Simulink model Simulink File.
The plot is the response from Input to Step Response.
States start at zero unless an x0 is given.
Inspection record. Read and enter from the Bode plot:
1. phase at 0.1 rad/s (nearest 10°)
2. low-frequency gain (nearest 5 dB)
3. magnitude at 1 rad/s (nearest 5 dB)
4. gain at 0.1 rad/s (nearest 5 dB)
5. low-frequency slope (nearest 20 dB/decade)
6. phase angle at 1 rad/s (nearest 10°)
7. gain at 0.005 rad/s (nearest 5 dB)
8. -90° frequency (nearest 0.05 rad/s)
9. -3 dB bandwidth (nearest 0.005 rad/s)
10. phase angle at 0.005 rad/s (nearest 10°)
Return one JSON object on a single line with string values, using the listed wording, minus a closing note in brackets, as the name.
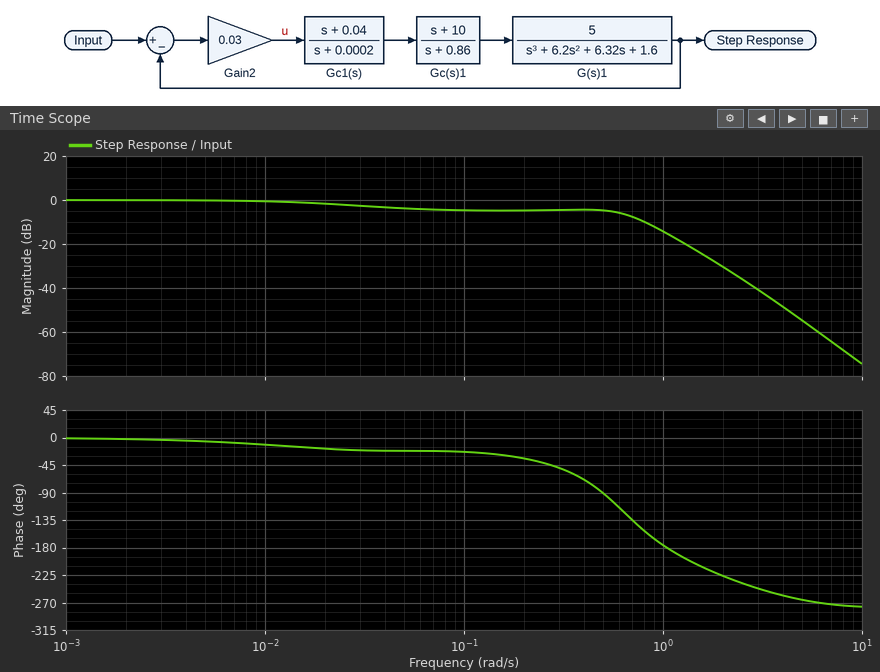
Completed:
{"phase at 0.1 rad/s": "-20°", "low-frequency gain": "0 dB", "magnitude at 1 rad/s": "-15 dB", "gain at 0.1 rad/s": "-5 dB", "low-frequency slope": "0 dB/decade", "phase angle at 1 rad/s": "-180°", "gain at 0.005 rad/s": "0 dB", "-90° frequency": "0.50 rad/s", "-3 dB bandwidth": "0.035 rad/s", "phase angle at 0.005 rad/s": "-10°"}
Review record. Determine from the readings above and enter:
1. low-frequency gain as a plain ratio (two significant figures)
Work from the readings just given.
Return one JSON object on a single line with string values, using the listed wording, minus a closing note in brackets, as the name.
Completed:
{"low-frequency gain as a plain ratio": "1.0"}
